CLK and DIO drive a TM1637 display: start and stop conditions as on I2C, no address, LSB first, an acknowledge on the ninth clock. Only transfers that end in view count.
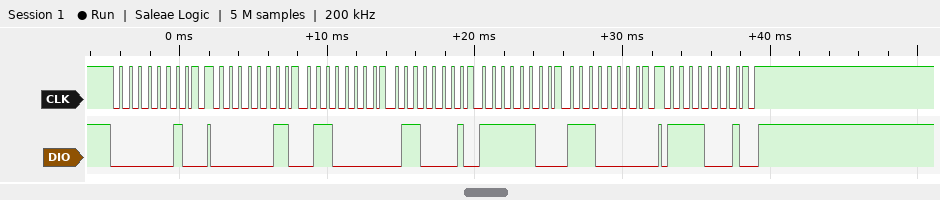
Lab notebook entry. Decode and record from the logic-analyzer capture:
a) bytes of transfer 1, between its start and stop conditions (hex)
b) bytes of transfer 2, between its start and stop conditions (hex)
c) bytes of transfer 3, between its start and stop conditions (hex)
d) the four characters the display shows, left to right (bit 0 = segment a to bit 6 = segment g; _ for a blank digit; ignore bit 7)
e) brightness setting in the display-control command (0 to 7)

40
C0 06 86 3F 07
8F
1107
7
